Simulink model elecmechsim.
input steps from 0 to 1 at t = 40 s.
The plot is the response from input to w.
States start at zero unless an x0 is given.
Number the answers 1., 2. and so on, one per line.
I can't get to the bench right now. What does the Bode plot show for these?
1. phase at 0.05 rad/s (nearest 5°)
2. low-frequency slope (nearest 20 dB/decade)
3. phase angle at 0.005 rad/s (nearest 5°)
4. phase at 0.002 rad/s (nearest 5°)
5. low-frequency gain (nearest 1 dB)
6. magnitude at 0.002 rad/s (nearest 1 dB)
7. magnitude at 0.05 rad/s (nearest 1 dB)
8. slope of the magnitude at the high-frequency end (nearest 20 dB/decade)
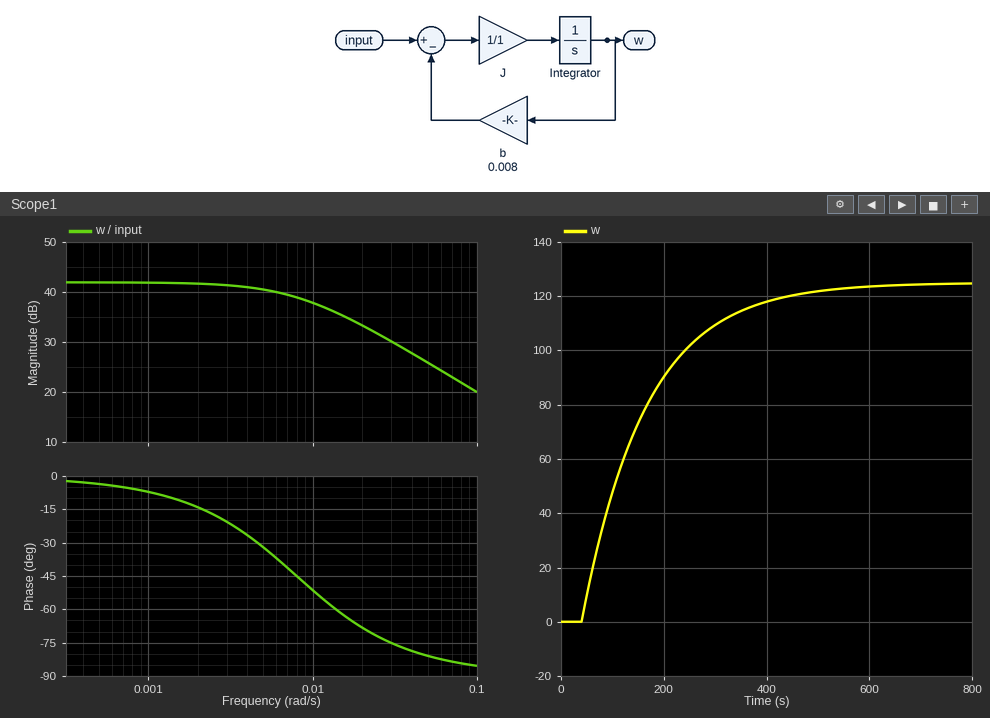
1. -80°
2. 0 dB/decade
3. -30°
4. -15°
5. 42 dB
6. 42 dB
7. 26 dB
8. -20 dB/decade
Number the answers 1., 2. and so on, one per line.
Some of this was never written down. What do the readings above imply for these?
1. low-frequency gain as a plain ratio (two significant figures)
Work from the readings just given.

1. 130
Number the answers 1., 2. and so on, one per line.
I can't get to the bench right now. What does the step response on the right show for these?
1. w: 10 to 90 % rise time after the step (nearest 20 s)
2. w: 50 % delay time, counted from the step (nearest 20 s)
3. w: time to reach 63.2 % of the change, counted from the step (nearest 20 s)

1. 280 s
2. 80 s
3. 120 s
